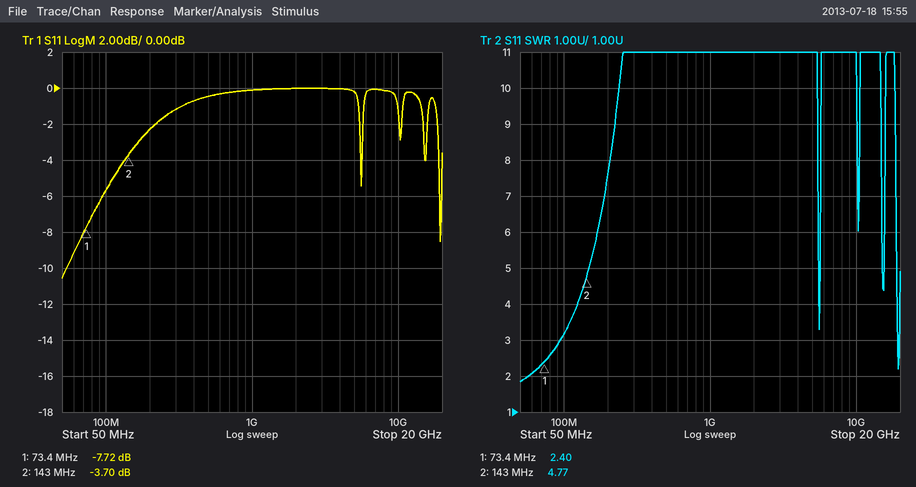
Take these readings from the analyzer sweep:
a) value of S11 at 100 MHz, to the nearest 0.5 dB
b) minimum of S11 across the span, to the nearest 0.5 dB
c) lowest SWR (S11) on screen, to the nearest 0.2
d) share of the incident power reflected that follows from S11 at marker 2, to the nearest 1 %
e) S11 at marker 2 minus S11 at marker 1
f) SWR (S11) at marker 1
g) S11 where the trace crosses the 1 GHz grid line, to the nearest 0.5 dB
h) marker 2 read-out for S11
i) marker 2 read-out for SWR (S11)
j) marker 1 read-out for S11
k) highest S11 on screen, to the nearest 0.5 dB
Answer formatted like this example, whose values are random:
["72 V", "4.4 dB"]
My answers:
["-5.5 dB", "-10.5 dB", "1.8", "43 %", "4.02 dB", "2.40", "0.0 dB", "-3.70 dB", "4.77", "-7.72 dB", "0.0 dB"]
